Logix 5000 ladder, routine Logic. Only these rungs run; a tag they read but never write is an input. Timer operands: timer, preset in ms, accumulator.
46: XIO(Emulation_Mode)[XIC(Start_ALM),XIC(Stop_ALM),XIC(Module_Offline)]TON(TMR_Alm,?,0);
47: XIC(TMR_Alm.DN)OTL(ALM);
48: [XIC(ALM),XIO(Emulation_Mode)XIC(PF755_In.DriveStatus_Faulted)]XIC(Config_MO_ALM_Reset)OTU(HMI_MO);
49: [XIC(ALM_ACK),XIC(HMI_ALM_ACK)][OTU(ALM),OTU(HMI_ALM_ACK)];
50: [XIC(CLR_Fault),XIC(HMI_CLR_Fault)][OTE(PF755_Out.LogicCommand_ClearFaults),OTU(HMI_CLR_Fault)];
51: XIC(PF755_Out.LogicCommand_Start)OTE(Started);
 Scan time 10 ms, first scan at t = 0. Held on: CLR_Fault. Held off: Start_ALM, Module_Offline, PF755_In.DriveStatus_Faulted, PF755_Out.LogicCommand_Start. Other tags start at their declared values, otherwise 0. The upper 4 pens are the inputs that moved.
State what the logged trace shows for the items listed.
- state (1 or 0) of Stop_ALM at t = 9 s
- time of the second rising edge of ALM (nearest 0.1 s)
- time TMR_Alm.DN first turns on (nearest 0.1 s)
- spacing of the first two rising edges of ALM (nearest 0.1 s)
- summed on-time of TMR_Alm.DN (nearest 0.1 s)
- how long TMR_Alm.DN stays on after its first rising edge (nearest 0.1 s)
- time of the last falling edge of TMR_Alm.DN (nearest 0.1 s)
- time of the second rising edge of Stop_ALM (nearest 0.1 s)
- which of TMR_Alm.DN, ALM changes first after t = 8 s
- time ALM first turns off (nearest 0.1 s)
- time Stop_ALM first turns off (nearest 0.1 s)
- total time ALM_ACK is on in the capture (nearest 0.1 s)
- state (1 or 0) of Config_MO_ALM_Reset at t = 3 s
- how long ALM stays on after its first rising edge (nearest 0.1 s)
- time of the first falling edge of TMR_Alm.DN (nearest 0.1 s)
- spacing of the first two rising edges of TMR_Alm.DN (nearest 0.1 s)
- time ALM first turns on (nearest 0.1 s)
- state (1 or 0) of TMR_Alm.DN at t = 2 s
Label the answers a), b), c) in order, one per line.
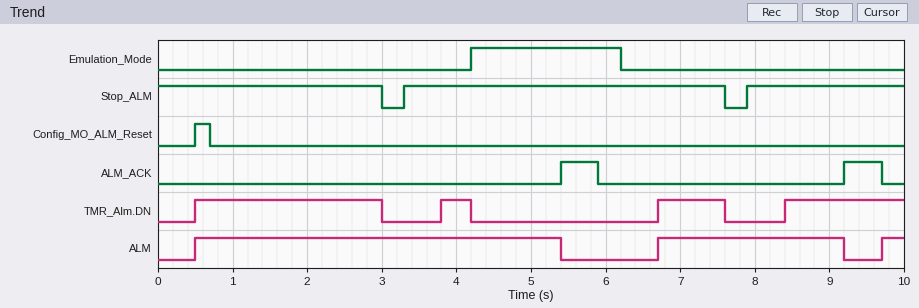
a) 1
b) 6.7 s
c) 0.5 s
d) 6.2 s
e) 5.4 s
f) 2.5 s
g) 7.6 s
h) 7.9 s
i) TMR_Alm.DN
j) 5.4 s
k) 3.0 s
l) 1.0 s
m) 0
n) 4.9 s
o) 3.0 s
p) 3.3 s
q) 0.5 s
r) 1
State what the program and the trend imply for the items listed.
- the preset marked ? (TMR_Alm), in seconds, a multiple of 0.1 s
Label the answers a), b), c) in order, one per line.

a) 0.5 s
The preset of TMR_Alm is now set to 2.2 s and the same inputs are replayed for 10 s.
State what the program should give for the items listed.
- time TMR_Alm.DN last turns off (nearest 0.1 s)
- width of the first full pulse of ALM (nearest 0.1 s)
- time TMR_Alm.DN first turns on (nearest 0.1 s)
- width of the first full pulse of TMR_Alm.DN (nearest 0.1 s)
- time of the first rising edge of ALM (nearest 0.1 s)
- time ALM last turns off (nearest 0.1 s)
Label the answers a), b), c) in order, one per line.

a) 3.0 s
b) 3.2 s
c) 2.2 s
d) 0.8 s
e) 2.2 s
f) 5.4 s
